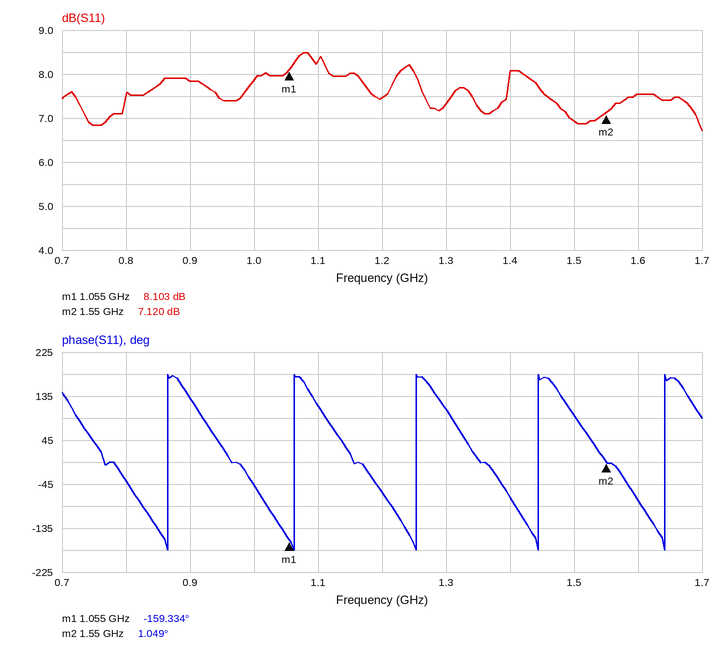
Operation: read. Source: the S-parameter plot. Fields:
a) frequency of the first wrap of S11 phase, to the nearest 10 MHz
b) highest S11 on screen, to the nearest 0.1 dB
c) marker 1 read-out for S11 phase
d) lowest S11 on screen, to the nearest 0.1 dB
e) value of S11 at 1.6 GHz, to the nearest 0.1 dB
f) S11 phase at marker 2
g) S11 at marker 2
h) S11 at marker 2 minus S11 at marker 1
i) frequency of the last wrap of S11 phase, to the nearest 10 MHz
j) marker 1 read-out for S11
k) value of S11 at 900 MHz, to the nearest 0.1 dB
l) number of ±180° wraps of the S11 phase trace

860 MHz
8.5 dB
-159.334°
6.7 dB
7.5 dB
1.049°
7.120 dB
-0.983 dB
1.64 GHz
8.103 dB
7.8 dB
5
